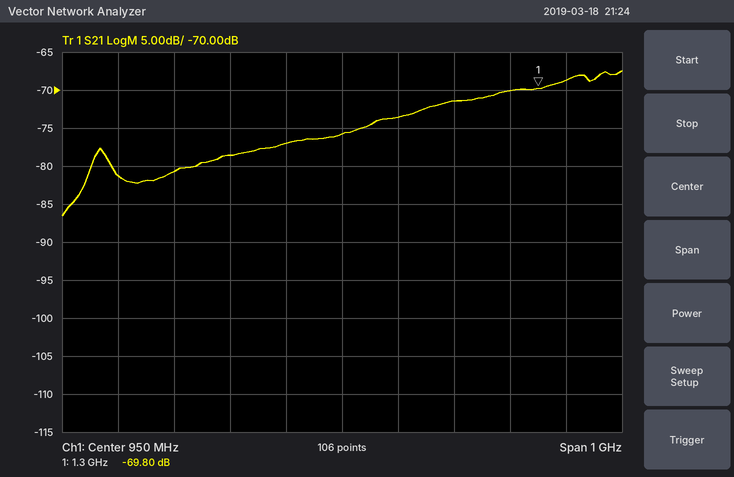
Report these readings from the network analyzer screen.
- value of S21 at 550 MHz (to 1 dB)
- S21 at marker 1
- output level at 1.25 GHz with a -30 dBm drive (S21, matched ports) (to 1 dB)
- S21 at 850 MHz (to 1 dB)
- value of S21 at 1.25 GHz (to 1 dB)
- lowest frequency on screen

-81 dB
-69.80 dB
-100 dBm
-77 dB
-70 dB
450 MHz
